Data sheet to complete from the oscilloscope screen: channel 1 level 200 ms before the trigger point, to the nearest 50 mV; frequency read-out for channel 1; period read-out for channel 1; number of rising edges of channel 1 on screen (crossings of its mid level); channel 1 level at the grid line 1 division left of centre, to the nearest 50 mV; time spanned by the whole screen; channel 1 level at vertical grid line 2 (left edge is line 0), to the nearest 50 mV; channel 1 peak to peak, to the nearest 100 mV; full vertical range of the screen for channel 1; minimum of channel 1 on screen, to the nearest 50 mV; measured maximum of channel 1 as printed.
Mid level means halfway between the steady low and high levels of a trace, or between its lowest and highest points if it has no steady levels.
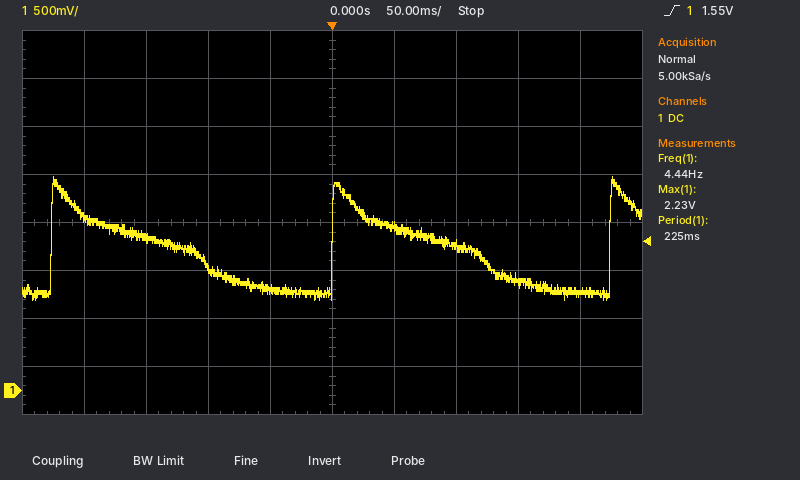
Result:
1.80 V
4.44 Hz
225 ms
3
1.05 V
500 ms
1.60 V
1.30 V
4 V
950 mV
2.23 V
